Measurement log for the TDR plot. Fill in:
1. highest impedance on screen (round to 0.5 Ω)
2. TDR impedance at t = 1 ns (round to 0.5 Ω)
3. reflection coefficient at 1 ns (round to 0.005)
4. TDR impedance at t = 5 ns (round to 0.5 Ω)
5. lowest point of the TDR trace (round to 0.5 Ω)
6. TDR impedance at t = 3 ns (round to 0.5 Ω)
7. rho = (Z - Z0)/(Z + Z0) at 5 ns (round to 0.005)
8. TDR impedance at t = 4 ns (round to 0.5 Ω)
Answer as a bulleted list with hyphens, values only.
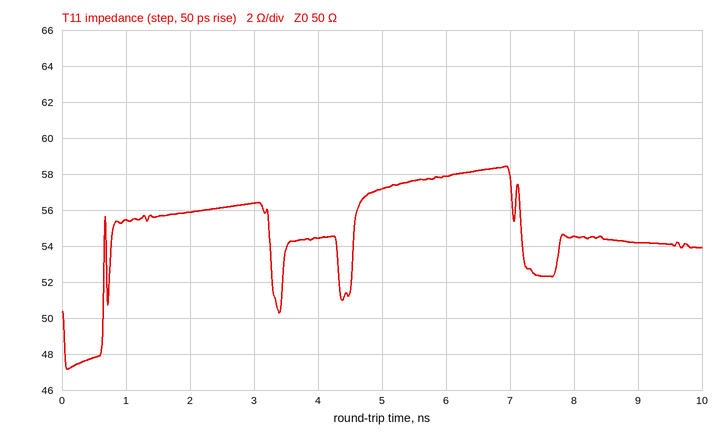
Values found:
- 58.5 Ω
- 55.5 Ω
- +0.050
- 57.0 Ω
- 47.0 Ω
- 56.5 Ω
- +0.065
- 54.5 Ω
